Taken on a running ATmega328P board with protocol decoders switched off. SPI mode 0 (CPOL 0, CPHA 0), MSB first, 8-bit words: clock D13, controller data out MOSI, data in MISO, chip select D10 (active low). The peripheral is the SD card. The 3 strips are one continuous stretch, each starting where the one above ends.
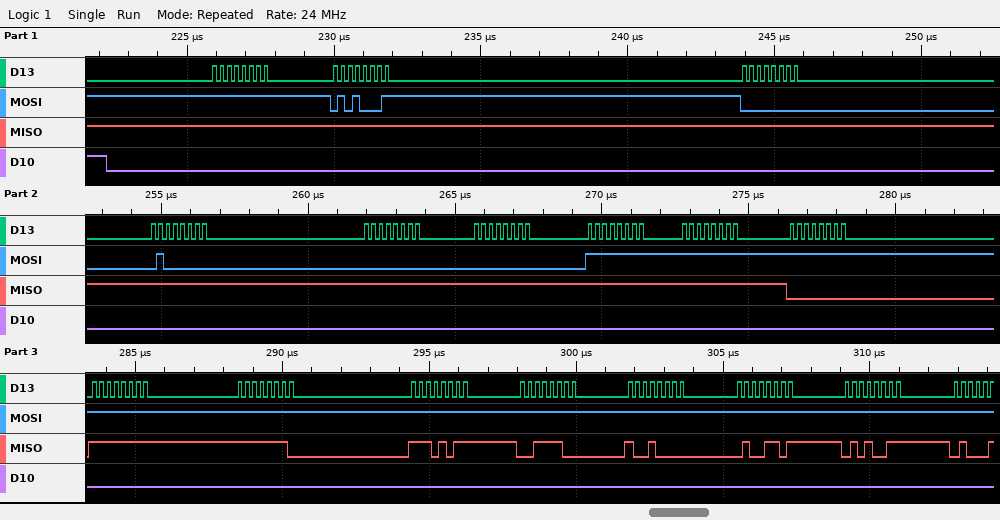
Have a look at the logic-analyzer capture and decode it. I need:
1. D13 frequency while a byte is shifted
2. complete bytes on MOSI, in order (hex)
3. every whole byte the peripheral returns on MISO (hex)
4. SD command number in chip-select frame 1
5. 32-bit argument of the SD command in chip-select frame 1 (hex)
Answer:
4 MHz
0xFF 0x51 0x00 0x40 0x00 0x00 0xFF 0xFF 0xFF 0xFF 0xFF 0xFF 0xFF 0xFF 0xFF 0xFF
0xFF 0xFF 0xFF 0xFF 0xFF 0xFF 0xFF 0xFF 0x00 0xFF 0xFE 0xEB 0x3C 0x90 0x4D 0x53
CMD17
0x00400000
